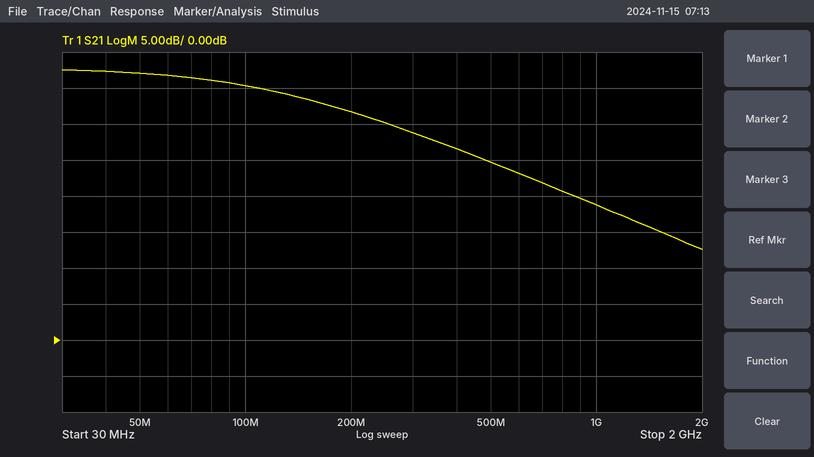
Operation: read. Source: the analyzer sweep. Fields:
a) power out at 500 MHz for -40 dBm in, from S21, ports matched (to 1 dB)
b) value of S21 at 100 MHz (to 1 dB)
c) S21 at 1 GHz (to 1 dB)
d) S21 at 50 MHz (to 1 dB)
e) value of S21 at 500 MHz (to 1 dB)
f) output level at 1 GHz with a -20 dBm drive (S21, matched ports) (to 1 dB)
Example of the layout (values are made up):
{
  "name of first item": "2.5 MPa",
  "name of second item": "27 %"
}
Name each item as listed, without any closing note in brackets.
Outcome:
{
  "power out at 500 MHz for -40 dBm in, from S21, ports matched": "-15 dBm",
  "value of S21 at 100 MHz": "35 dB",
  "S21 at 1 GHz": "19 dB",
  "S21 at 50 MHz": "37 dB",
  "value of S21 at 500 MHz": "25 dB",
  "output level at 1 GHz with a -20 dBm drive (S21, matched ports)": "-1 dBm"
}
